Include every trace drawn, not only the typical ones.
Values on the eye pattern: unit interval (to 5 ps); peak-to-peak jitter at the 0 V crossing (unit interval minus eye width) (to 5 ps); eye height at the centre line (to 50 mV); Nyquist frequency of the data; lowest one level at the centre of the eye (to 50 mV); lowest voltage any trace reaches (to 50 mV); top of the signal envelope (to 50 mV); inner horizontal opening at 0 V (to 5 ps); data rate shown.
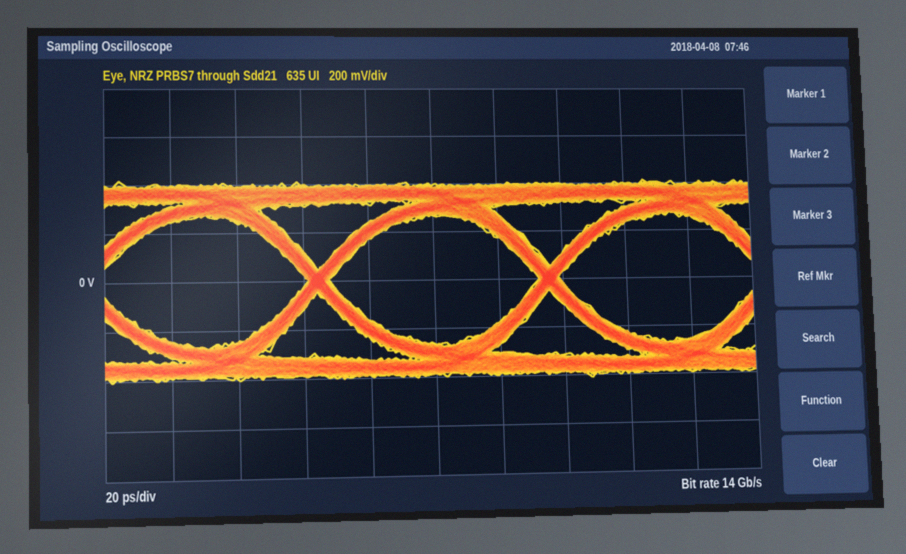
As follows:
70 ps
5 ps
550 mV
7 GHz
250 mV
-400 mV
400 mV
65 ps
14 Gb/s
